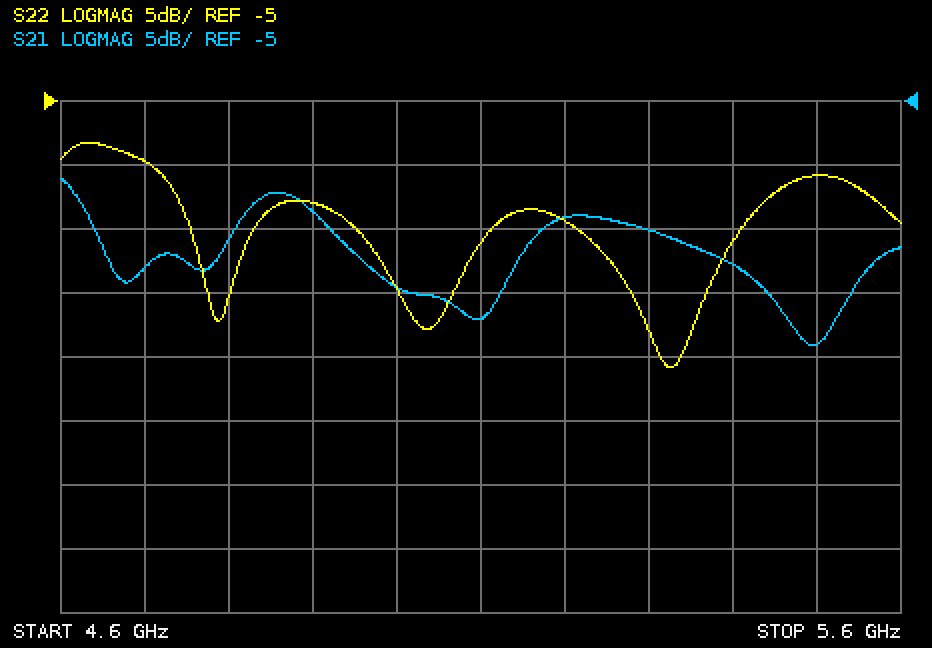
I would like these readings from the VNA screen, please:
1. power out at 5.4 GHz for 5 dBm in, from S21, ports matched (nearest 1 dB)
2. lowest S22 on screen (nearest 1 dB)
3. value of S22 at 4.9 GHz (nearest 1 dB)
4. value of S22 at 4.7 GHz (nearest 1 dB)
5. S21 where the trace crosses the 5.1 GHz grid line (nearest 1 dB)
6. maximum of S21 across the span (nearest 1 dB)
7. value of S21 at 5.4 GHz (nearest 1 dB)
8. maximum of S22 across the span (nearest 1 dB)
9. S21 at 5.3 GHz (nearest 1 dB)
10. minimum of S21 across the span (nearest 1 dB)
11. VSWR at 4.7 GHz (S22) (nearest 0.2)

-13 dBm
-26 dB
-13 dB
-10 dB
-22 dB
-11 dB
-18 dB
-8 dB
-15 dB
-24 dB
2.0
